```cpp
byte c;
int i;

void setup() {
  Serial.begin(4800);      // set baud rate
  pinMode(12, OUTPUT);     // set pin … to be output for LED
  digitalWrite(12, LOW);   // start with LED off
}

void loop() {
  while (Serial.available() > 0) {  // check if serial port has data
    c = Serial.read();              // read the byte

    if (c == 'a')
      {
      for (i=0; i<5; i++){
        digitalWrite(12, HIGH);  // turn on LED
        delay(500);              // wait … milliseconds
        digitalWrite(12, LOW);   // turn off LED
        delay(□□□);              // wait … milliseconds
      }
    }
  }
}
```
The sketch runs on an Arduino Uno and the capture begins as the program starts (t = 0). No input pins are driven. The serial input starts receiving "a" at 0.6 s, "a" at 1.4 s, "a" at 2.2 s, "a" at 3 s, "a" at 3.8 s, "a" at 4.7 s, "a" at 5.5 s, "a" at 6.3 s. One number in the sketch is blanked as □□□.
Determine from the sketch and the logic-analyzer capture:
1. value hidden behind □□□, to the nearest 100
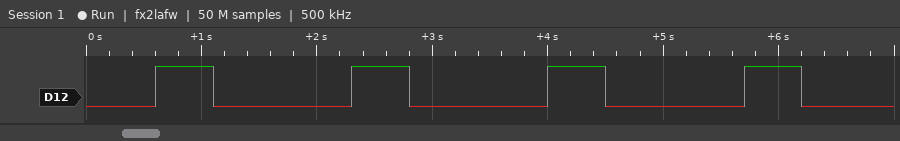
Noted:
1200
